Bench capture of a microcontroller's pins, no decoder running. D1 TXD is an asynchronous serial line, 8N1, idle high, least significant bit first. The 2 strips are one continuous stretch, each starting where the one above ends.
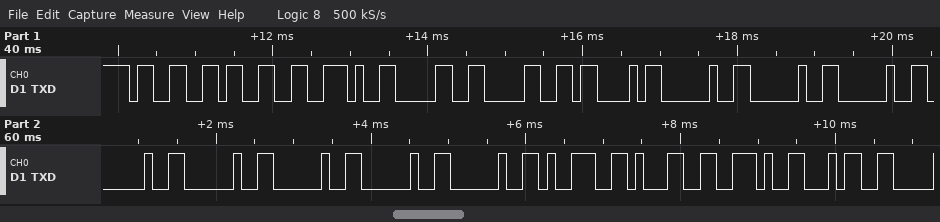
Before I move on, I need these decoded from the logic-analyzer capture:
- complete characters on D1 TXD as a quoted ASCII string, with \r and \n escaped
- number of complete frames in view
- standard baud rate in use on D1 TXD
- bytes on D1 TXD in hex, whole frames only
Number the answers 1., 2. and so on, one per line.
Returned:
1. "33.00C        91.4"
2. 18
3. 9600 baud
4. 33 33 2E 30 30 43 20 20 20 20 20 20 20 20 39 31 2E 34
